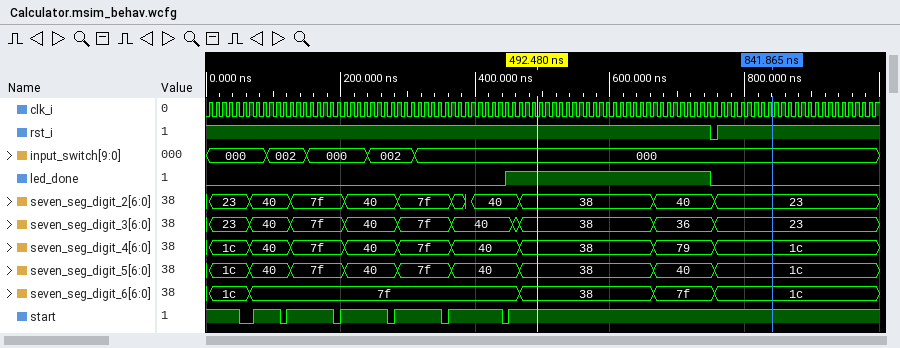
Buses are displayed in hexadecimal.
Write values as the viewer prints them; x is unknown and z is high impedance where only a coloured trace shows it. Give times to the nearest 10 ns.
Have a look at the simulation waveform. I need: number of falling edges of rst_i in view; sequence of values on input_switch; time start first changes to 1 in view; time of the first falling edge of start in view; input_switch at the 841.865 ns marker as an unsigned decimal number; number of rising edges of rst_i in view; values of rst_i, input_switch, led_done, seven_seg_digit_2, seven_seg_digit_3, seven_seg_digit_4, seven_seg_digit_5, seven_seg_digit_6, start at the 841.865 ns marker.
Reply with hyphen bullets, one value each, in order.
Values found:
- 1
- 000, 002, 000, 002, 000
- 70 ns
- 50 ns
- 0
- 1
- rst_i=1, input_switch=000, led_done=0, seven_seg_digit_2=23, seven_seg_digit_3=23, seven_seg_digit_4=1c, seven_seg_digit_5=1c, seven_seg_digit_6=1c, start=1
